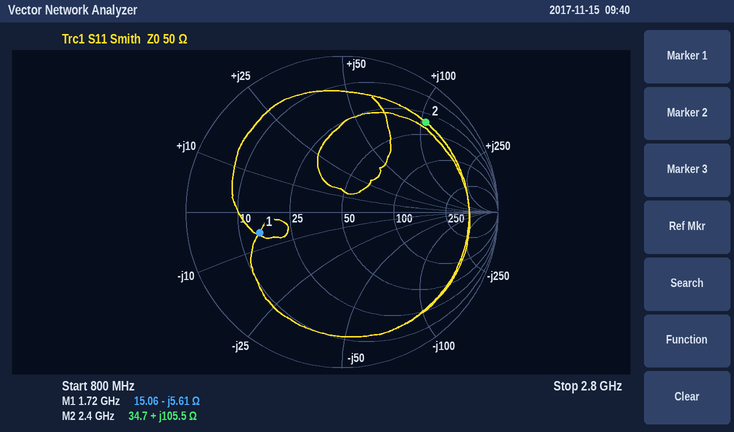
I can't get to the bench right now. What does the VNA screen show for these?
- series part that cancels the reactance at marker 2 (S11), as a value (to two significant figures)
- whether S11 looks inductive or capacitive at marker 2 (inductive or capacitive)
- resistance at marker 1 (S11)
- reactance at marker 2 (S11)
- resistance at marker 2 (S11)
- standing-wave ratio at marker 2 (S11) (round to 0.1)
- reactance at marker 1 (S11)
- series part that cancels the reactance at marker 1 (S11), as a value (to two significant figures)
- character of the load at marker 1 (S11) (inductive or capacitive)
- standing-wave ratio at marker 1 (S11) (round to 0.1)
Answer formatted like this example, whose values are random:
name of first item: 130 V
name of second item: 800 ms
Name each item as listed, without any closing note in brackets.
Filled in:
series part that cancels the reactance at marker 2 (S11), as a value: 630 fF
whether S11 looks inductive or capacitive at marker 2: inductive
resistance at marker 1: 15.06 Ω
reactance at marker 2: +105.5 Ω
resistance at marker 2: 34.7 Ω
standing-wave ratio at marker 2 (S11): 8.4
reactance at marker 1: -5.61 Ω
series part that cancels the reactance at marker 1 (S11), as a value: 520 pH
character of the load at marker 1 (S11): capacitive
standing-wave ratio at marker 1 (S11): 3.4
